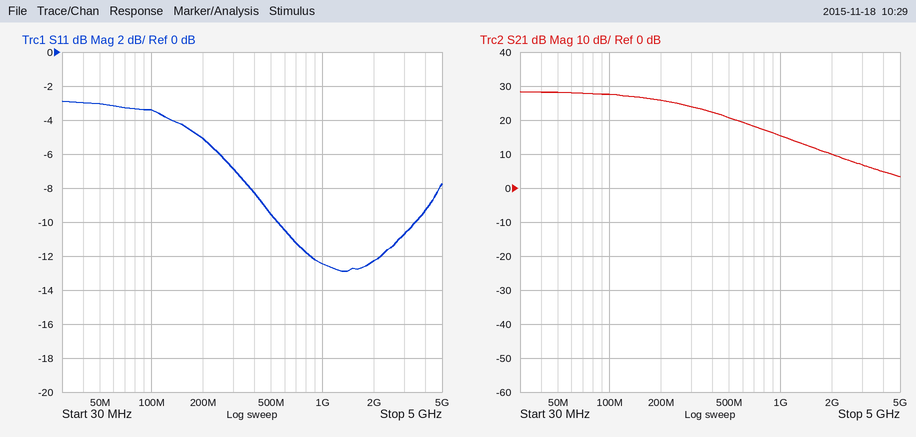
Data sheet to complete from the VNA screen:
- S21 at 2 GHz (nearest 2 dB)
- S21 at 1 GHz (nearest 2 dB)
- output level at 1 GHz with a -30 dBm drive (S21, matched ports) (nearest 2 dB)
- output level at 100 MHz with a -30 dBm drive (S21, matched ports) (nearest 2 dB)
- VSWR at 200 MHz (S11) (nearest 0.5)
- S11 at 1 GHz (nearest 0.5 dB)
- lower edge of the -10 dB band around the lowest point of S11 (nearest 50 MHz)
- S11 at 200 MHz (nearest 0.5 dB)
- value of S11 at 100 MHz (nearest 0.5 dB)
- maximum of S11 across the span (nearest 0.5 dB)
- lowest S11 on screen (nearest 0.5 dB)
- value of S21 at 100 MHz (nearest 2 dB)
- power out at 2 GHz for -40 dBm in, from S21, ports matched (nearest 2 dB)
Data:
10 dB
16 dB
-14 dBm
-2 dBm
3.5
-12.5 dB
550 MHz
-5.0 dB
-3.5 dB
-3.0 dB
-13.0 dB
28 dB
-30 dBm
